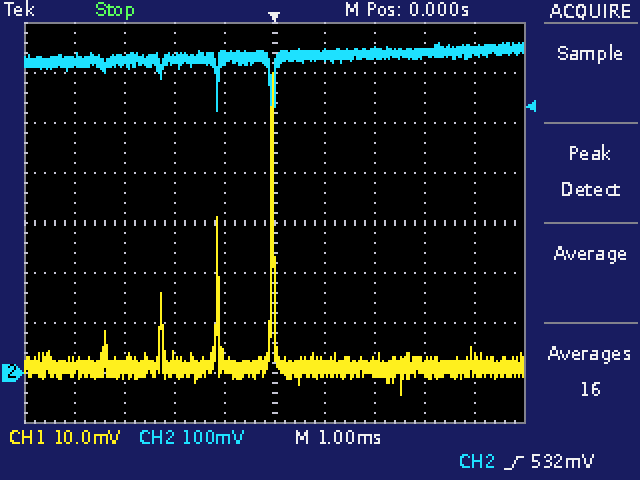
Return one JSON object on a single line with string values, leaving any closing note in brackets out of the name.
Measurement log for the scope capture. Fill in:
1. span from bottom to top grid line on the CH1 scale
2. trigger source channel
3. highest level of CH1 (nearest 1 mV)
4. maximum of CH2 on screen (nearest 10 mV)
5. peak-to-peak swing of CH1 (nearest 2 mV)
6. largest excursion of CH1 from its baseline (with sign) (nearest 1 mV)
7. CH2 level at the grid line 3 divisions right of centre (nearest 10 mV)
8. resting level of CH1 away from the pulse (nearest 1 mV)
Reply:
{"span from bottom to top grid line on the CH1 scale": "80 mV", "trigger source channel": "CH2", "highest level of CH1": "60 mV", "maximum of CH2 on screen": "660 mV", "peak-to-peak swing of CH1": "64 mV", "largest excursion of CH1 from its baseline (with sign)": "+59 mV", "CH2 level at the grid line 3 divisions right of centre": "640 mV", "resting level of CH1 away from the pulse": "1 mV"}
